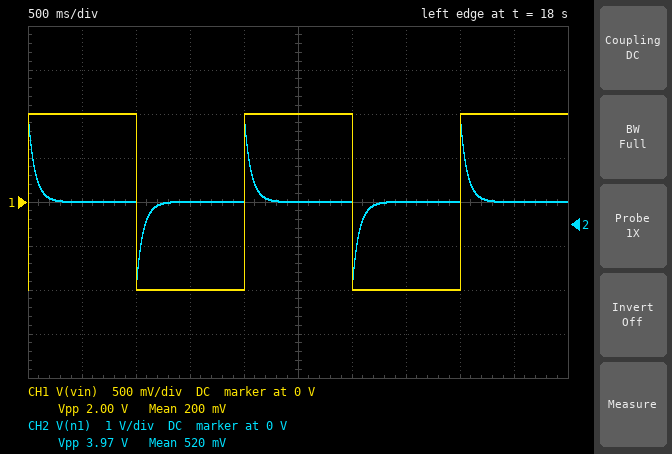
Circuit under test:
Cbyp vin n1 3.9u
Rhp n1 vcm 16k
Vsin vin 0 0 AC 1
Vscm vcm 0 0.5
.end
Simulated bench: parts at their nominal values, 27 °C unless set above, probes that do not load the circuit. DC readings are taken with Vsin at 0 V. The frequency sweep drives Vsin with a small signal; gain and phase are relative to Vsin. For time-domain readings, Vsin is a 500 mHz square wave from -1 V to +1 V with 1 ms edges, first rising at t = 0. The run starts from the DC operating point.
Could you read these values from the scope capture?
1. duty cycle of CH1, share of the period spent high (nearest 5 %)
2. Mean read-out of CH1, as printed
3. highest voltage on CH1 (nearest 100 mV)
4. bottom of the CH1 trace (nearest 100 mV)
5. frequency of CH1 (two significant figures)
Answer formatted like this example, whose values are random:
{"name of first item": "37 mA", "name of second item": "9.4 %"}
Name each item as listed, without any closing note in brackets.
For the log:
{"duty cycle of CH1, share of the period spent high": "50 %", "Mean read-out of CH1, as printed": "200 mV", "highest voltage on CH1": "1.0 V", "bottom of the CH1 trace": "-1.0 V", "frequency of CH1": "500 mHz"}
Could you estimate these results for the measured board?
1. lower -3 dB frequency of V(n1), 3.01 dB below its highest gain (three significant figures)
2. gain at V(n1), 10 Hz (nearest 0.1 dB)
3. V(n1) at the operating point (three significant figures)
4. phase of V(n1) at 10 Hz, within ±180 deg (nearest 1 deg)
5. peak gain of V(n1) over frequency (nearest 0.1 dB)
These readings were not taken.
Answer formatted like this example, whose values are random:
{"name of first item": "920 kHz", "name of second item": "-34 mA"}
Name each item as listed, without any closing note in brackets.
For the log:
{"lower -3 dB frequency of V(n1), 3.01 dB below its highest gain": "2.55 Hz", "gain at V(n1), 10 Hz": "-0.3 dB", "V(n1) at the operating point": "500 mV", "phase of V(n1) at 10 Hz, within ±180 deg": "14 deg", "peak gain of V(n1) over frequency": "0 dB"}
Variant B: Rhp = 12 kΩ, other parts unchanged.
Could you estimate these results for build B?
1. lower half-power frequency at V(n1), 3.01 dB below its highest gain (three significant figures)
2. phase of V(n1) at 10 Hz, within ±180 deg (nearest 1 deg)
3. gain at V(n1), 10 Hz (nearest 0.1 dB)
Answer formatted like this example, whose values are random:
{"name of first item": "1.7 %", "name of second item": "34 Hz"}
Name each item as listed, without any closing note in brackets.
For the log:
{"lower half-power frequency at V(n1), 3.01 dB below its highest gain": "3.40 Hz", "phase of V(n1) at 10 Hz, within ±180 deg": "19 deg", "gain at V(n1), 10 Hz": "-0.5 dB"}
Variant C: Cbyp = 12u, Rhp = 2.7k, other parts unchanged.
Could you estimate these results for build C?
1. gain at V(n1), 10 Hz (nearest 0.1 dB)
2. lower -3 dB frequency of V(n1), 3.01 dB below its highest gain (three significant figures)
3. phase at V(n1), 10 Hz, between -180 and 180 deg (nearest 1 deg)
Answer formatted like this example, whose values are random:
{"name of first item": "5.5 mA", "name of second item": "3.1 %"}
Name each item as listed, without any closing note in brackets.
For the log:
{"gain at V(n1), 10 Hz": "-0.9 dB", "lower -3 dB frequency of V(n1), 3.01 dB below its highest gain": "4.91 Hz", "phase at V(n1), 10 Hz, between -180 and 180 deg": "26 deg"}
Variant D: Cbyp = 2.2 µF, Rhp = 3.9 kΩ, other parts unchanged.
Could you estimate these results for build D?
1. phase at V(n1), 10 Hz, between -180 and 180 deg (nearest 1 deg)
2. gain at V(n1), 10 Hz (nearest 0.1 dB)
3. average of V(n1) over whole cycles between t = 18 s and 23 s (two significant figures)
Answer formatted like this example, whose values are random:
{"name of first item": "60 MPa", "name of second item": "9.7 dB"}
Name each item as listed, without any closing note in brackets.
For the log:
{"phase at V(n1), 10 Hz, between -180 and 180 deg": "62 deg", "gain at V(n1), 10 Hz": "-6.5 dB", "average of V(n1) over whole cycles between t = 18 s and 23 s": "500 mV"}
